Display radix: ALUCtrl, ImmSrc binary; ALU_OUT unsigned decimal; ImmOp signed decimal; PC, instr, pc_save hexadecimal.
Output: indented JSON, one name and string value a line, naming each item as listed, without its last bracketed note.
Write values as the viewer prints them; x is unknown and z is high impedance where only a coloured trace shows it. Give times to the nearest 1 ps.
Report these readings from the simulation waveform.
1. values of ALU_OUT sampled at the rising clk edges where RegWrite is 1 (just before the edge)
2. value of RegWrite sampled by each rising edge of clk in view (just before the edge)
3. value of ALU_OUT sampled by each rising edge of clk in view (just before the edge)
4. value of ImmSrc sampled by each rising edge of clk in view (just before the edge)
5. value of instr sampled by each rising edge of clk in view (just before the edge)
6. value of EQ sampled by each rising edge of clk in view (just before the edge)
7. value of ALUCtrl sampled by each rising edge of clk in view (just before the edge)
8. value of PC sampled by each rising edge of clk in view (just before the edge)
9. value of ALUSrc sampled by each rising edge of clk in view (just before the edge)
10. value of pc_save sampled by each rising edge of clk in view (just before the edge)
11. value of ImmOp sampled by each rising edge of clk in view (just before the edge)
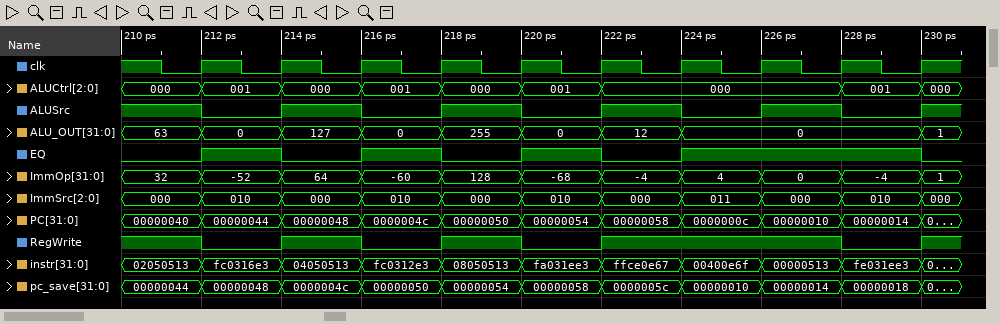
{
  "values of ALU_OUT sampled at the rising clk edges where RegWrite is 1": "63, 127, 255, 12, 0, 0",
  "value of RegWrite sampled by each rising edge of clk in view": "1 0 1 0 1 0 1 1 1 0",
  "value of ALU_OUT sampled by each rising edge of clk in view": "63, 0, 127, 0, 255, 0, 12, 0, 0, 0",
  "value of ImmSrc sampled by each rising edge of clk in view": "000, 010, 000, 010, 000, 010, 000, 011, 000, 010",
  "value of instr sampled by each rising edge of clk in view": "02050513, fc0316e3, 04050513, fc0312e3, 08050513, fa031ee3, ffce0e67, 00400e6f, 00000513, fe031ee3",
  "value of EQ sampled by each rising edge of clk in view": "0 1 0 1 0 1 0 1 1 1",
  "value of ALUCtrl sampled by each rising edge of clk in view": "000, 001, 000, 001, 000, 001, 000, 000, 000, 001",
  "value of PC sampled by each rising edge of clk in view": "00000040, 00000044, 00000048, 0000004c, 00000050, 00000054, 00000058, 0000000c, 00000010, 00000014",
  "value of ALUSrc sampled by each rising edge of clk in view": "1 0 1 0 1 0 1 0 1 0",
  "value of pc_save sampled by each rising edge of clk in view": "00000044, 00000048, 0000004c, 00000050, 00000054, 00000058, 0000005c, 00000010, 00000014, 00000018",
  "value of ImmOp sampled by each rising edge of clk in view": "32, -52, 64, -60, 128, -68, -4, 4, 0, -4"
}
